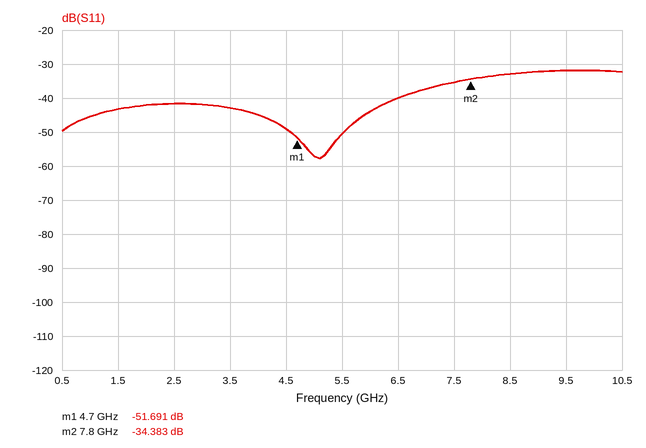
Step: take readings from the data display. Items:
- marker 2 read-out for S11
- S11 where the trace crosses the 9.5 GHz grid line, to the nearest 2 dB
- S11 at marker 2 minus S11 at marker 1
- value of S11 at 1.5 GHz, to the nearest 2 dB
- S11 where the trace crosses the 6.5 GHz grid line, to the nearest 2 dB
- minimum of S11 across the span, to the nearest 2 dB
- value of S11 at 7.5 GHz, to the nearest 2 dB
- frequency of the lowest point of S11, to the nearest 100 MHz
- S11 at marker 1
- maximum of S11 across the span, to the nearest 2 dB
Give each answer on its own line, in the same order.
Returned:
-34.383 dB
-32 dB
17.308 dB
-44 dB
-40 dB
-58 dB
-36 dB
5.1 GHz
-51.691 dB
-32 dB
